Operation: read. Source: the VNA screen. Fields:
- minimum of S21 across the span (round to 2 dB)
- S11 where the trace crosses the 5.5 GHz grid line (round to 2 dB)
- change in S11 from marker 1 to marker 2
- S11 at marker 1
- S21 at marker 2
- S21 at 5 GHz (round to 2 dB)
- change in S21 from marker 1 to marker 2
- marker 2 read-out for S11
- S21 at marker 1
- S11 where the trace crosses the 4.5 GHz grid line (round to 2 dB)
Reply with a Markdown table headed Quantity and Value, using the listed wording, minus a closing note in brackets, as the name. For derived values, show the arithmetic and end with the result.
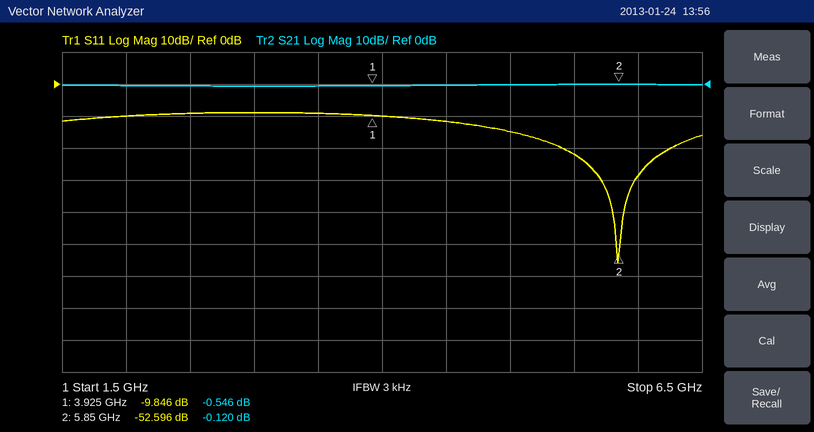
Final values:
| Quantity | Value |
|---|---|
| minimum of S21 across the span | 0 dB |
| S11 where the trace crosses the 5.5 GHz grid line | -22 dB |
| change in S11 from marker 1 to marker 2 | -52.596 − (-9.846) = -42.750 dB |
| S11 at marker 1 | -9.846 dB |
| S21 at marker 2 | -0.120 dB |
| S21 at 5 GHz | 0 dB |
| change in S21 from marker 1 to marker 2 | -0.12 − (-0.546) = 0.426 dB |
| marker 2 read-out for S11 | -52.596 dB |
| S21 at marker 1 | -0.546 dB |
| S11 where the trace crosses the 4.5 GHz grid line | -12 dB |
